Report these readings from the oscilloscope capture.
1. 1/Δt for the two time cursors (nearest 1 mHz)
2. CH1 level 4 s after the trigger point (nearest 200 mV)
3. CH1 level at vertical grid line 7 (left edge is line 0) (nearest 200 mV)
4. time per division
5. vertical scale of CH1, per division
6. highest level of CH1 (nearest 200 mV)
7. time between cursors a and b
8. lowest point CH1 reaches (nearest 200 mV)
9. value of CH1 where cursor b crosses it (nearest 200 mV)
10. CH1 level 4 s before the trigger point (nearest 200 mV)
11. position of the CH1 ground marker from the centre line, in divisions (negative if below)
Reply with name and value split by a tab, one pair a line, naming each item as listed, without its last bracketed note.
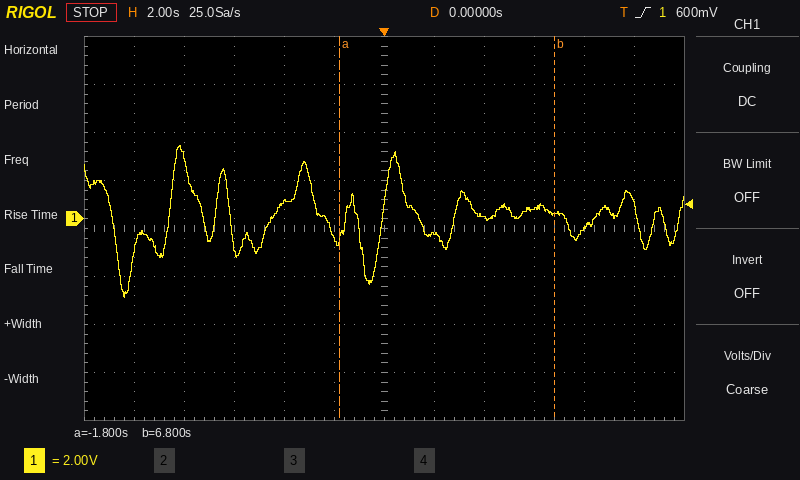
1/Δt for the two time cursors	116 mHz
CH1 level 4 s after the trigger point	0.0 V
CH1 level at vertical grid line 7 (left edge is line 0)	-600 mV
time per division	2 s
vertical scale of CH1, per division	2 V
highest level of CH1	3.0 V
time between cursors a and b	8.6 s
lowest point CH1 reaches	-3.2 V
value of CH1 where cursor b crosses it	200 mV
CH1 level 4 s before the trigger point	600 mV
position of the CH1 ground marker from the centre line, in divisions	+0.2 div
